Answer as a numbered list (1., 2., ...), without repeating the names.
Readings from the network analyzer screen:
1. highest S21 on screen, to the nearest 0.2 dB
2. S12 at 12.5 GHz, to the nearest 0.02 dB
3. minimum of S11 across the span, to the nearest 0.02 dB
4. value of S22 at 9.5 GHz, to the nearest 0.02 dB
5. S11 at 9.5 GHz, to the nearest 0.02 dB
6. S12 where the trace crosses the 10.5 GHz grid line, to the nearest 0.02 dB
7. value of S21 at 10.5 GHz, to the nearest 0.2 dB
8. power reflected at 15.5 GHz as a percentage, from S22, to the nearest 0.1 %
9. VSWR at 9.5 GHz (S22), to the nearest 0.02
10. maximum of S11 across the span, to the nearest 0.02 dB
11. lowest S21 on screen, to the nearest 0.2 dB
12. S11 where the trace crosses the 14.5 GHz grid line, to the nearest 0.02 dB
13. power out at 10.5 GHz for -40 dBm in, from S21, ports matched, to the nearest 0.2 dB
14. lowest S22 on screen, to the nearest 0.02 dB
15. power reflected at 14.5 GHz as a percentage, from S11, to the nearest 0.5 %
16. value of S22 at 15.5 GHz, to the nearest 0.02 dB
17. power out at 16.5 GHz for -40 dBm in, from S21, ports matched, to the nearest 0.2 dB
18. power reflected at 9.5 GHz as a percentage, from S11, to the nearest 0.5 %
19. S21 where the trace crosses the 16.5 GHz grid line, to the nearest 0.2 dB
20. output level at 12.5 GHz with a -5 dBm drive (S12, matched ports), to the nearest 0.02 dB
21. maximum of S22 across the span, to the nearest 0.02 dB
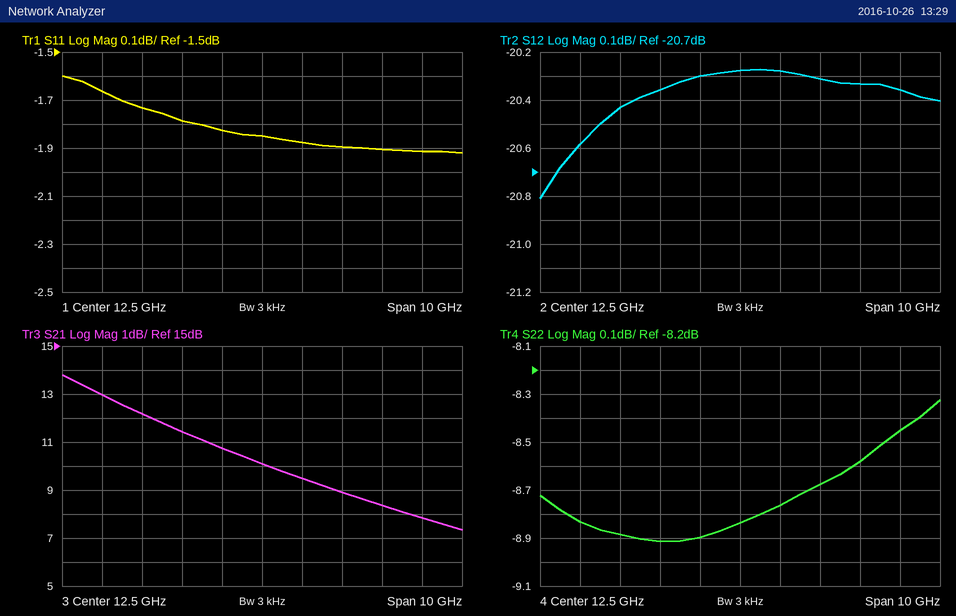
1. 13.8 dB
2. -20.28 dB
3. -1.92 dB
4. -8.88 dB
5. -1.74 dB
6. -20.36 dB
7. 11.4 dB
8. 13.9 %
9. 2.12
10. -1.60 dB
11. 7.4 dB
12. -1.90 dB
13. -28.6 dBm
14. -8.92 dB
15. 64.5 %
16. -8.58 dB
17. -32.2 dBm
18. 67.0 %
19. 7.8 dB
20. -25.28 dBm
21. -8.32 dB
